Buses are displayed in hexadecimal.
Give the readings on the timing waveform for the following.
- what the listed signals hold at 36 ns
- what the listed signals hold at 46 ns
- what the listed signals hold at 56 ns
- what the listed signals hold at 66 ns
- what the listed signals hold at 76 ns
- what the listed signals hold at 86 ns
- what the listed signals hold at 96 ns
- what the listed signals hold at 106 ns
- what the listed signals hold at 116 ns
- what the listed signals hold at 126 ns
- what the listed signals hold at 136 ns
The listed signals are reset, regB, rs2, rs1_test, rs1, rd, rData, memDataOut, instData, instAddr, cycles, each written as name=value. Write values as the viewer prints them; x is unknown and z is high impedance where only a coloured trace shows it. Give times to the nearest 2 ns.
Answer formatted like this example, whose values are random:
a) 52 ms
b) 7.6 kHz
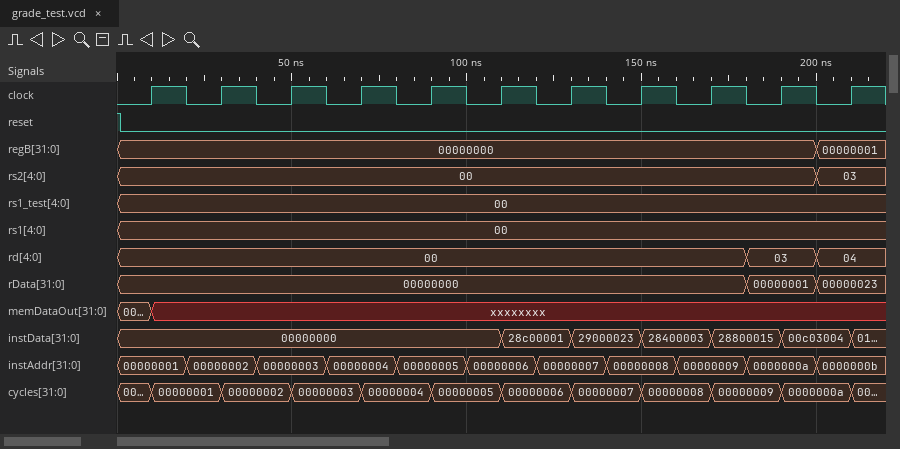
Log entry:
a) reset=0, regB=00000000, rs2=00, rs1_test=00, rs1=00, rd=00, rData=00000000, memDataOut=xxxxxxxx, instData=00000000, instAddr=00000002, cycles=00000002
b) reset=0, regB=00000000, rs2=00, rs1_test=00, rs1=00, rd=00, rData=00000000, memDataOut=xxxxxxxx, instData=00000000, instAddr=00000003, cycles=00000002
c) reset=0, regB=00000000, rs2=00, rs1_test=00, rs1=00, rd=00, rData=00000000, memDataOut=xxxxxxxx, instData=00000000, instAddr=00000003, cycles=00000003
d) reset=0, regB=00000000, rs2=00, rs1_test=00, rs1=00, rd=00, rData=00000000, memDataOut=xxxxxxxx, instData=00000000, instAddr=00000004, cycles=00000003
e) reset=0, regB=00000000, rs2=00, rs1_test=00, rs1=00, rd=00, rData=00000000, memDataOut=xxxxxxxx, instData=00000000, instAddr=00000004, cycles=00000004
f) reset=0, regB=00000000, rs2=00, rs1_test=00, rs1=00, rd=00, rData=00000000, memDataOut=xxxxxxxx, instData=00000000, instAddr=00000005, cycles=00000004
g) reset=0, regB=00000000, rs2=00, rs1_test=00, rs1=00, rd=00, rData=00000000, memDataOut=xxxxxxxx, instData=00000000, instAddr=00000005, cycles=00000005
h) reset=0, regB=00000000, rs2=00, rs1_test=00, rs1=00, rd=00, rData=00000000, memDataOut=xxxxxxxx, instData=00000000, instAddr=00000006, cycles=00000005
i) reset=0, regB=00000000, rs2=00, rs1_test=00, rs1=00, rd=00, rData=00000000, memDataOut=xxxxxxxx, instData=28c00001, instAddr=00000006, cycles=00000006
j) reset=0, regB=00000000, rs2=00, rs1_test=00, rs1=00, rd=00, rData=00000000, memDataOut=xxxxxxxx, instData=28c00001, instAddr=00000007, cycles=00000006
k) reset=0, regB=00000000, rs2=00, rs1_test=00, rs1=00, rd=00, rData=00000000, memDataOut=xxxxxxxx, instData=29000023, instAddr=00000007, cycles=00000007
